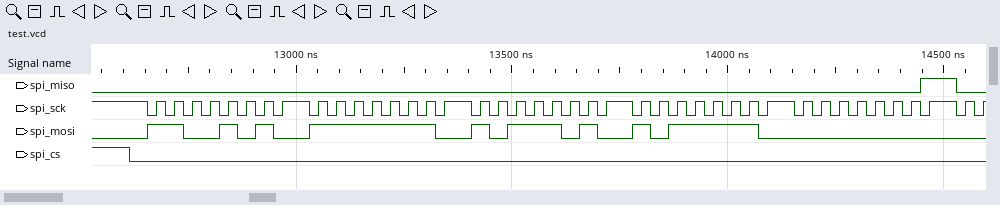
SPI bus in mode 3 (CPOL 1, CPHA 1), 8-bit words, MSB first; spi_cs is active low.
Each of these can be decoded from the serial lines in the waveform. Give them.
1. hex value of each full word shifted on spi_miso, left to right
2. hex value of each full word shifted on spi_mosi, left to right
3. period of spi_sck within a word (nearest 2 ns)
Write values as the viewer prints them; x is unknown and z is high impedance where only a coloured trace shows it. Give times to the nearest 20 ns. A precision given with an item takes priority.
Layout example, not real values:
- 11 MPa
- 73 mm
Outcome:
- 00, 00, 00, 00, 01
- CA, FE, BA, BE, 00
- 42 ns
